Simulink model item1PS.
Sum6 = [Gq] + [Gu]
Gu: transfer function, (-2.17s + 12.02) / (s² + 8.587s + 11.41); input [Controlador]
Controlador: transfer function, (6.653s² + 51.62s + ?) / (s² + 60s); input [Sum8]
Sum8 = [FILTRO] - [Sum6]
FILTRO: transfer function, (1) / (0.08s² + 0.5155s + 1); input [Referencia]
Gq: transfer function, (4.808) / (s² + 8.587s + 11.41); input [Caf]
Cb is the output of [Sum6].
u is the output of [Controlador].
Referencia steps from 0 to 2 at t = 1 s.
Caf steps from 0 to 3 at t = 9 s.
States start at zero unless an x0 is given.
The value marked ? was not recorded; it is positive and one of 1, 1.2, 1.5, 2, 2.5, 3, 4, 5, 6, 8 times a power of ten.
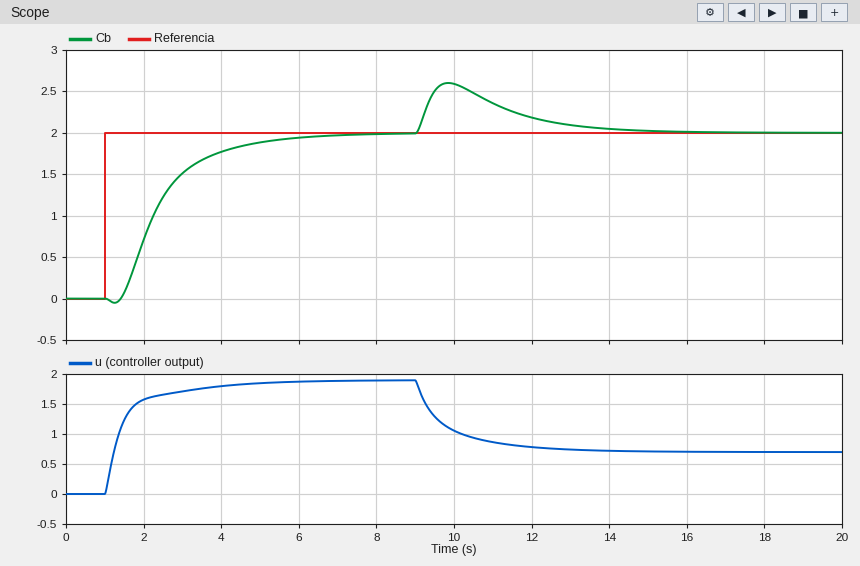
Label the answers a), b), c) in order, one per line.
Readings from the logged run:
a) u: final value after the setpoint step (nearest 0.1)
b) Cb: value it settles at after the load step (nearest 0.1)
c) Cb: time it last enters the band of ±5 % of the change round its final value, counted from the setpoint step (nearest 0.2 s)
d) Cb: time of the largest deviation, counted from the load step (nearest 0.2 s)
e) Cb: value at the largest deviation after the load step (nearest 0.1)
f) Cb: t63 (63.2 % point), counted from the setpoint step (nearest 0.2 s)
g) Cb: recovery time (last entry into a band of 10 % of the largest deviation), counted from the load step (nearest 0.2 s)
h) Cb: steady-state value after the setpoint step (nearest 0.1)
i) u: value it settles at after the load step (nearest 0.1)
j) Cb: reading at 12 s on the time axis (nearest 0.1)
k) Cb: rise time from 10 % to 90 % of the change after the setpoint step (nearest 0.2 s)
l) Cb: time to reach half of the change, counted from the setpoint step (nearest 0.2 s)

a) 1.9
b) 2.0
c) 4.2 s
d) 0.8 s
e) 2.6
f) 1.6 s
g) 4.6 s
h) 2.0
i) 0.7
j) 2.2
k) 2.6 s
l) 1.2 s
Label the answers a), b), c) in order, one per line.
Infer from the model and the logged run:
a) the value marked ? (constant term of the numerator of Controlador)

a) 50
